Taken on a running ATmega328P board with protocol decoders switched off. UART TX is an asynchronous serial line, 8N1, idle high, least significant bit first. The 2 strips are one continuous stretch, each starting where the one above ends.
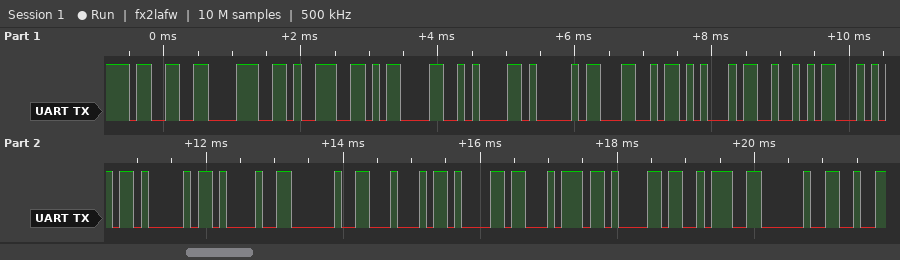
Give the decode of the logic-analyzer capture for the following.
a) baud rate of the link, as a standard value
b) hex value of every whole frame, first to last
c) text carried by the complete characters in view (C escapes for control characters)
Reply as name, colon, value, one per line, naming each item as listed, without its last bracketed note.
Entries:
baud rate of the link, as a standard value: 9600 baud
hex value of every whole frame, first to last: 33 38 39 0D 0A 41 4C 45 52 54 41 21 20 44 61 74 61 3A 20
text carried by the complete characters in view: "389\r\nALERTA! Data: "
